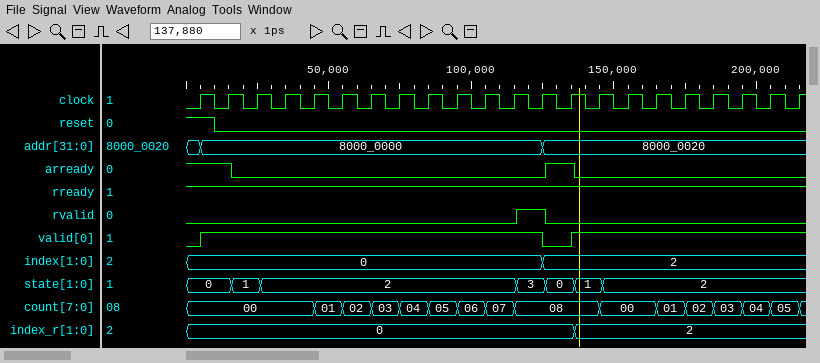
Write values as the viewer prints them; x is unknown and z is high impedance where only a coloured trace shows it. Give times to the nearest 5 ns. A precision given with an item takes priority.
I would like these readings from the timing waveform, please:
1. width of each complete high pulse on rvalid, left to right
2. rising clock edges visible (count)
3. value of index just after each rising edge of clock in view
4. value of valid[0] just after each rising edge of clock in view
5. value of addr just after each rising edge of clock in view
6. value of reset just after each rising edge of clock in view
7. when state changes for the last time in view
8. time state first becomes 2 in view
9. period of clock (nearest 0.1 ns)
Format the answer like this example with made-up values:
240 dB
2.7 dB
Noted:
10 ns
22
0, 0, 0, 0, 0, 0, 0, 0, 0, 0, 0, 0, 2, 2, 2, 2, 2, 2, 2, 2, 2, 2
1 1 1 1 1 1 1 1 1 1 1 1 0 1 1 1 1 1 1 1 1 1
8000_0000, 8000_0000, 8000_0000, 8000_0000, 8000_0000, 8000_0000, 8000_0000, 8000_0000, 8000_0000, 8000_0000, 8000_0000, 8000_0000, 8000_0020, 8000_0020, 8000_0020, 8000_0020, 8000_0020, 8000_0020, 8000_0020, 8000_0020, 8000_0020, 8000_0020
1 0 0 0 0 0 0 0 0 0 0 0 0 0 0 0 0 0 0 0 0 0
145 ns
25 ns
10 ns
